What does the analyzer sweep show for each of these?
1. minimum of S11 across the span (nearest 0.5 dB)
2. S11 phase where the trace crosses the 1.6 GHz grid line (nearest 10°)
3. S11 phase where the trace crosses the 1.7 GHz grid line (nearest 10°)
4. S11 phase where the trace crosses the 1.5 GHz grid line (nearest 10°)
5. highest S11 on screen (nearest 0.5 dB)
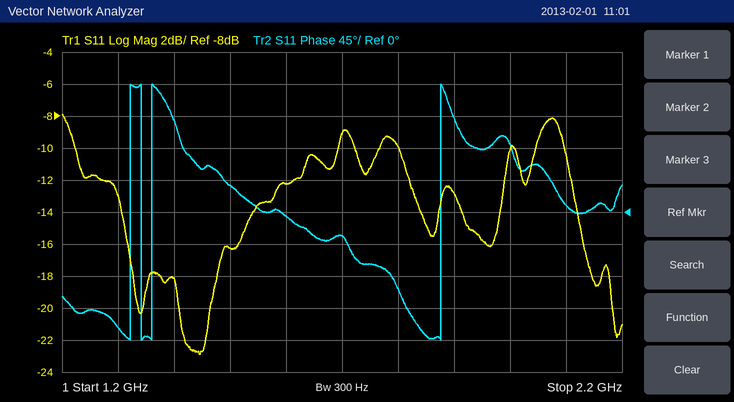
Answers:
-23.0 dB
-10°
-30°
40°
-8.0 dB
